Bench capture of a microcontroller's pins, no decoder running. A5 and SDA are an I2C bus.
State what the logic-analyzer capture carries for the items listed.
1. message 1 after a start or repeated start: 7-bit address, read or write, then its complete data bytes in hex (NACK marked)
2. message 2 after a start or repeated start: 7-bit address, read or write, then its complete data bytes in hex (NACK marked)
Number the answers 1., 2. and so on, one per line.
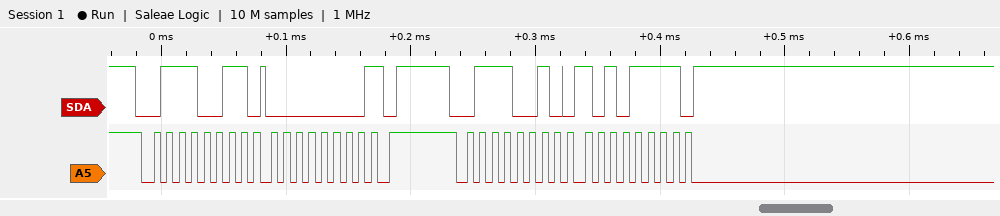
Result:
1. 0x39 read: 00 NACK
2. 0x39 write: AF
